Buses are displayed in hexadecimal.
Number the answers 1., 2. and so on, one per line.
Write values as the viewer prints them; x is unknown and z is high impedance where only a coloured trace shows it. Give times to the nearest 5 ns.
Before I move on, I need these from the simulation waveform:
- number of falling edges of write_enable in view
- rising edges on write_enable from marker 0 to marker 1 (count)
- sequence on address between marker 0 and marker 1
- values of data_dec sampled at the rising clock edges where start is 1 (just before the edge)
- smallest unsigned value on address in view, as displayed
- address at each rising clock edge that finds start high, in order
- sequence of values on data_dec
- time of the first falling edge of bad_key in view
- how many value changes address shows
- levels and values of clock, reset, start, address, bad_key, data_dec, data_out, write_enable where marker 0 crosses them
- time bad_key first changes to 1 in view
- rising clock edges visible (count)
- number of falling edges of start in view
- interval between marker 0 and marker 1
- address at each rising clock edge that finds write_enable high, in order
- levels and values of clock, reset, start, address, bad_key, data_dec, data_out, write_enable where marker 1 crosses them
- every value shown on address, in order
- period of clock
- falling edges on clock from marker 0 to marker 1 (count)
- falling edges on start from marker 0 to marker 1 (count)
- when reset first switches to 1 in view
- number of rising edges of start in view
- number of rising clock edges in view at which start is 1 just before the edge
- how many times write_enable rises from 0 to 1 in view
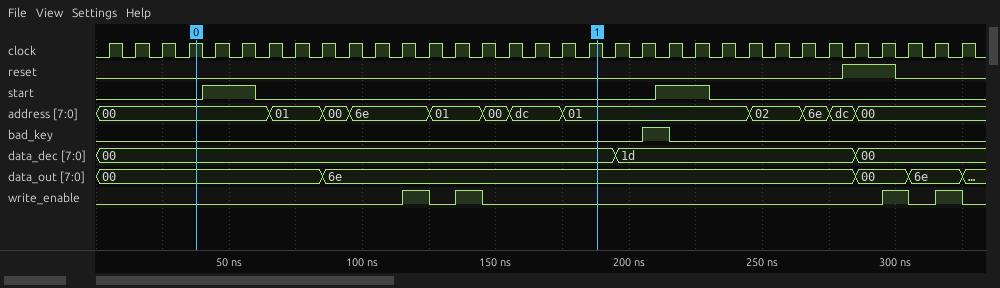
1. 4
2. 2
3. 00, 01, 00, 6e, 01, 00, dc, 01
4. 00, 00, 1d, 1d
5. 00
6. 00, 00, 01, 01
7. 00, 1d, 00
8. 215 ns
9. 11
10. clock=1, reset=0, start=0, address=00, bad_key=0, data_dec=00, data_out=00, write_enable=0
11. 205 ns
12. 33
13. 2
14. 150 ns
15. 6e, 01, 00, 00
16. clock=1, reset=0, start=0, address=01, bad_key=0, data_dec=00, data_out=6e, write_enable=0
17. 00, 01, 00, 6e, 01, 00, dc, 01, 02, 6e, dc, 00
18. 10 ns
19. 15
20. 1
21. 280 ns
22. 2
23. 4
24. 4
